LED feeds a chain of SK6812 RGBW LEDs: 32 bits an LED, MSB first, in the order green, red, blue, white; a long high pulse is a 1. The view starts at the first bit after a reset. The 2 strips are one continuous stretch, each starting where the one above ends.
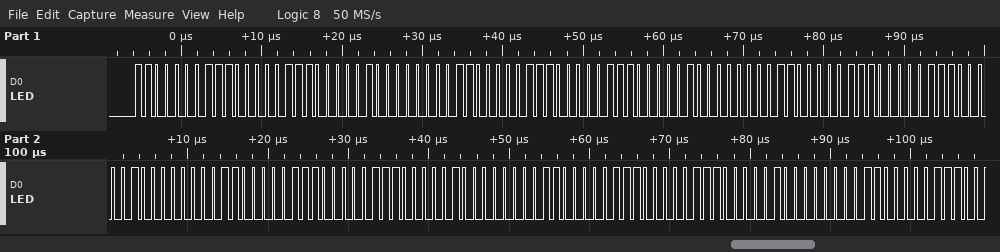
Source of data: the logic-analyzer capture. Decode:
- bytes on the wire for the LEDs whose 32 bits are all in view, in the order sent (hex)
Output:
C1 C1 C1 00 C1 C1 C1 00 C1 C1 C1 00 C1 C1 C1 00 C1 C1 C1 00
